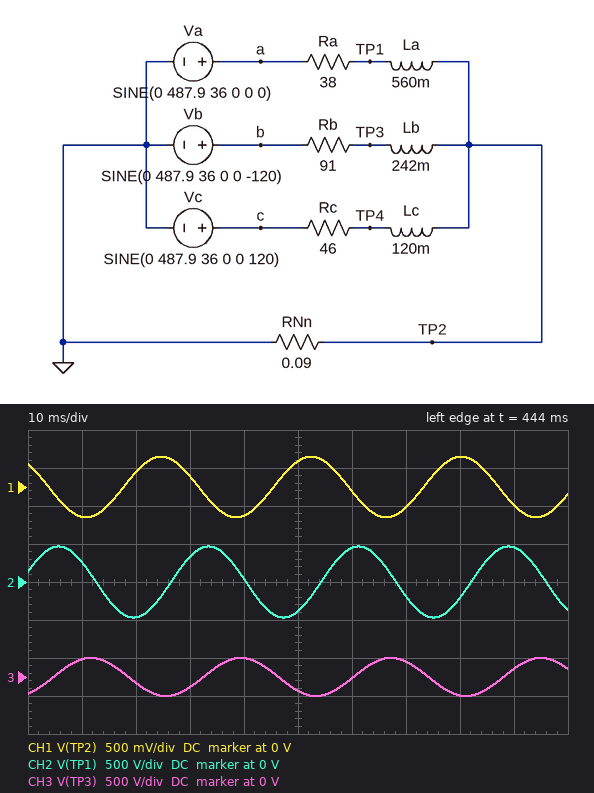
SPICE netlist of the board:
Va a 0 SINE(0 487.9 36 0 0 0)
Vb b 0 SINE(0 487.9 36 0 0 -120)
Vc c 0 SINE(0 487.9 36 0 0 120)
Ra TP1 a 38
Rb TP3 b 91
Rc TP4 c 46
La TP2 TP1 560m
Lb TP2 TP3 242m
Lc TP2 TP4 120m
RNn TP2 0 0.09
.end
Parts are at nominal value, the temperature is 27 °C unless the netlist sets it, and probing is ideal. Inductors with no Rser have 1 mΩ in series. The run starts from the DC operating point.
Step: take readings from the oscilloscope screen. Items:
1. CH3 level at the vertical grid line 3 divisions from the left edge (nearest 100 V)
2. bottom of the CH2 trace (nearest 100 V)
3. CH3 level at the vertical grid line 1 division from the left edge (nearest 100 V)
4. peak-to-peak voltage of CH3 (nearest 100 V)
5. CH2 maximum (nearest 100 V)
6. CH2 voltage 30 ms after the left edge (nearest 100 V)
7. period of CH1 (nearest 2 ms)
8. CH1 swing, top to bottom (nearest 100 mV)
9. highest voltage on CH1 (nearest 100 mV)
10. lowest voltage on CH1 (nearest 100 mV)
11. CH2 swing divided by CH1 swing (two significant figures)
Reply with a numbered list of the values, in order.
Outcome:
1. -100 V
2. -500 V
3. 200 V
4. 500 V
5. 500 V
6. 300 V
7. 28 ms
8. 800 mV
9. 400 mV
10. -400 mV
11. 1200
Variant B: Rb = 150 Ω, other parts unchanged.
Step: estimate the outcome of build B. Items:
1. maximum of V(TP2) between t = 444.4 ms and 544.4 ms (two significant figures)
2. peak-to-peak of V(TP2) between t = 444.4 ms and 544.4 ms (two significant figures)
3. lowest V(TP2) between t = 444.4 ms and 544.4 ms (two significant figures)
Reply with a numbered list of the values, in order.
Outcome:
1. 340 mV
2. 690 mV
3. -340 mV
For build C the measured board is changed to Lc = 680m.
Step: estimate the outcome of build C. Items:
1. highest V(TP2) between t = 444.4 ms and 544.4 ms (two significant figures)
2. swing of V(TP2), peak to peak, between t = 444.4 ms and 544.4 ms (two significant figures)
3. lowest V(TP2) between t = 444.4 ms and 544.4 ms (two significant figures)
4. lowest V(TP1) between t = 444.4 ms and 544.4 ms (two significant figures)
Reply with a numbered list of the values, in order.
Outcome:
1. 330 mV
2. 660 mV
3. -330 mV
4. -470 V
